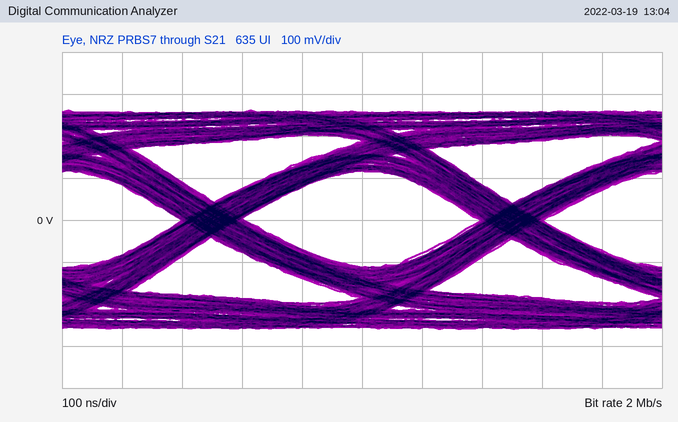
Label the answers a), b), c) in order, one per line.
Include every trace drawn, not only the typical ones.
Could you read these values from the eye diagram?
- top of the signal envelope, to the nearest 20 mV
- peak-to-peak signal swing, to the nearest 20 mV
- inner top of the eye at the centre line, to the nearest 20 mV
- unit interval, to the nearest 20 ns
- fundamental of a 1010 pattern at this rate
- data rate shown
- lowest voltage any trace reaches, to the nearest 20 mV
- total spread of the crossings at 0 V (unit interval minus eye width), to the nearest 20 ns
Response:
a) 260 mV
b) 520 mV
c) 120 mV
d) 500 ns
e) 1 MHz
f) 2 Mb/s
g) -260 mV
h) 100 ns
